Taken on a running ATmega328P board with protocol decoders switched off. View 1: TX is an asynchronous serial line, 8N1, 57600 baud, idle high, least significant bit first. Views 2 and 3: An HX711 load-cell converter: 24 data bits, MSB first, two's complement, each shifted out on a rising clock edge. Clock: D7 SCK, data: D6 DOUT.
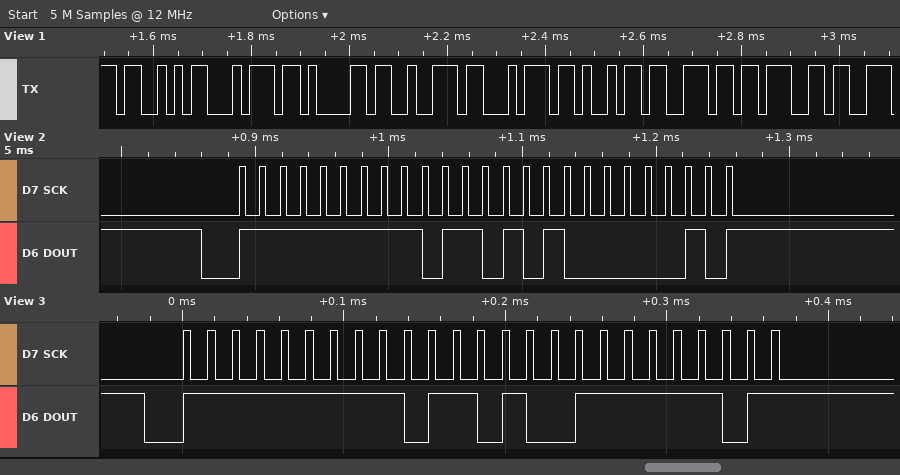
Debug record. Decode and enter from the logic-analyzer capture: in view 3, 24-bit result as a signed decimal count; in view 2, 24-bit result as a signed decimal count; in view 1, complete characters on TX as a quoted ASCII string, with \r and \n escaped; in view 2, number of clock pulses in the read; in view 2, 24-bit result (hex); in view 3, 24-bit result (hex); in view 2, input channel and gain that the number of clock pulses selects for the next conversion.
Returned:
-19203
-19198
"Starting"
25
0xFFB502
0xFFB4FD
channel A, gain 128
